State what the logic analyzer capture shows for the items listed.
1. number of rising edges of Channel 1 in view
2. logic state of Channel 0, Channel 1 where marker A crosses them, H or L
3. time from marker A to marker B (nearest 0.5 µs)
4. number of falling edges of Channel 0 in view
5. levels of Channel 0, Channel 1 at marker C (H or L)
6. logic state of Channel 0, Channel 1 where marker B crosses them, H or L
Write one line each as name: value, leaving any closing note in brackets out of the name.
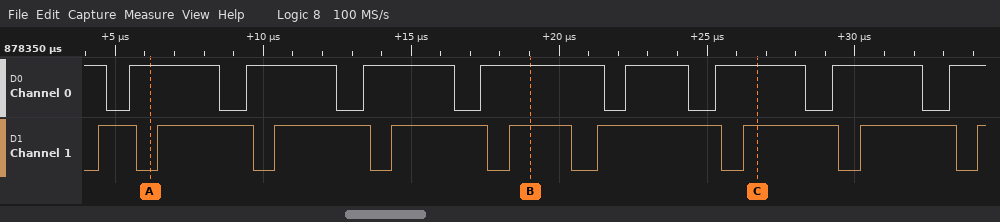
number of rising edges of Channel 1 in view: 9
logic state of Channel 0, Channel 1 where marker A crosses them, H or L: Channel 0=H, Channel 1=L
time from marker A to marker B: 13 µs
number of falling edges of Channel 0 in view: 8
levels of Channel 0, Channel 1 at marker C: Channel 0=H, Channel 1=H
logic state of Channel 0, Channel 1 where marker B crosses them, H or L: Channel 0=H, Channel 1=H
